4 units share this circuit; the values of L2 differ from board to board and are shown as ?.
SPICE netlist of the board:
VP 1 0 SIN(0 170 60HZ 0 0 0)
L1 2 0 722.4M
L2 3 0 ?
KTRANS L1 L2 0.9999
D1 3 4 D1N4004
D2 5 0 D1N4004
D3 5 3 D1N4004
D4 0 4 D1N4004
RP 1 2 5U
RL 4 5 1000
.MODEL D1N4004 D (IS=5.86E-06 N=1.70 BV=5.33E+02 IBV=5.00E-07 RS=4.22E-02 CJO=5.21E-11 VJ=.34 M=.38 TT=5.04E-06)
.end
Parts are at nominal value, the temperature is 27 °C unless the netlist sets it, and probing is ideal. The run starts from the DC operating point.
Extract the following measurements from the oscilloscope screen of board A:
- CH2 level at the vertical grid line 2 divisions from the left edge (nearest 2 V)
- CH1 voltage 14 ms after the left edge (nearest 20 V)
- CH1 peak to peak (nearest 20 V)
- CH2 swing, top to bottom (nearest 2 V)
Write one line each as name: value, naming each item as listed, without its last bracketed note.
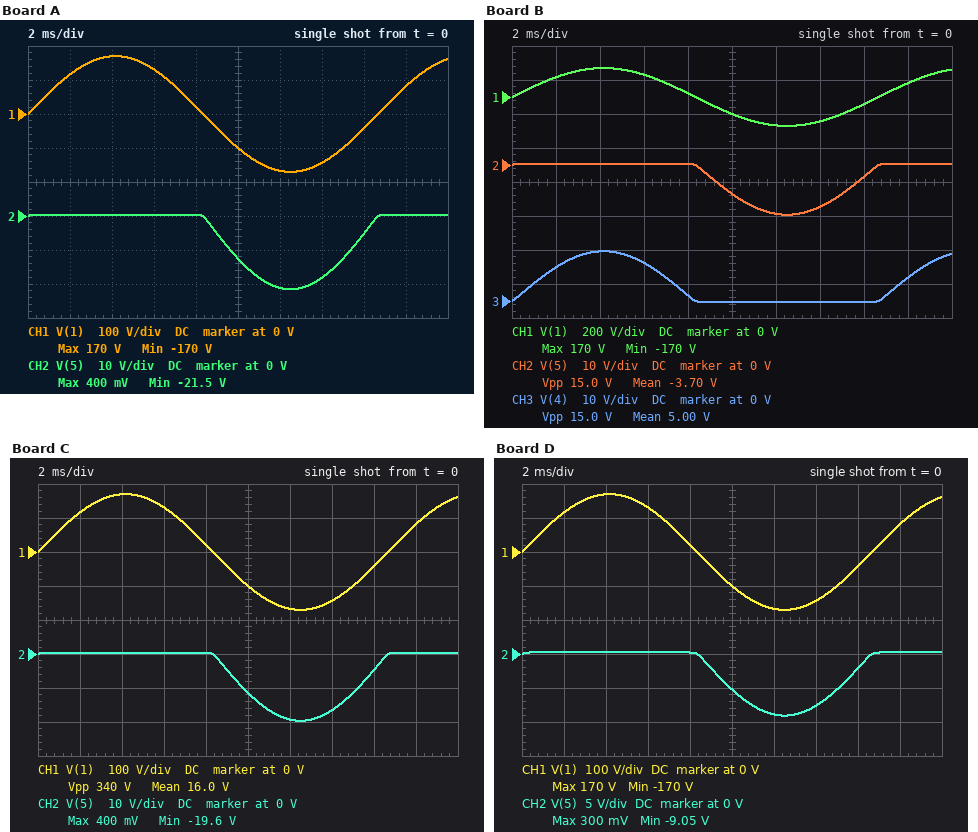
CH2 level at the vertical grid line 2 divisions from the left edge: 0 V
CH1 voltage 14 ms after the left edge: -140 V
CH1 peak to peak: 340 V
CH2 swing, top to bottom: 22 V
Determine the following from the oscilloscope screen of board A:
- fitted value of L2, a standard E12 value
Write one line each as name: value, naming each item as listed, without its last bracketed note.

fitted value of L2, a standard E12 value: 12 mH
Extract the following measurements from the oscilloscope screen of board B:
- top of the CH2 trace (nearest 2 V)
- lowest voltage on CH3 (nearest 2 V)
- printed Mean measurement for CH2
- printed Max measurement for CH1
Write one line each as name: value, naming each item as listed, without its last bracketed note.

top of the CH2 trace: 0 V
lowest voltage on CH3: 0 V
printed Mean measurement for CH2: -3.70 V
printed Max measurement for CH1: 170 V
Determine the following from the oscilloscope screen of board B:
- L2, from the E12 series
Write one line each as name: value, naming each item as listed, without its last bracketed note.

L2, from the E12 series: 5.6 mH
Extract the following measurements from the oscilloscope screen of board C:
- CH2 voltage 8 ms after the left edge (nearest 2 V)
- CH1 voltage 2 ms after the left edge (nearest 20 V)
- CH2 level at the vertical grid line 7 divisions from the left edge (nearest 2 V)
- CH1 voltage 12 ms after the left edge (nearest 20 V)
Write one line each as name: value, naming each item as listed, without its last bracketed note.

CH2 voltage 8 ms after the left edge: 0 V
CH1 voltage 2 ms after the left edge: 120 V
CH2 level at the vertical grid line 7 divisions from the left edge: -16 V
CH1 voltage 12 ms after the left edge: -160 V
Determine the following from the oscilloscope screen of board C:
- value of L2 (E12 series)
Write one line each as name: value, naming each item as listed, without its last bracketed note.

value of L2: 10 mH
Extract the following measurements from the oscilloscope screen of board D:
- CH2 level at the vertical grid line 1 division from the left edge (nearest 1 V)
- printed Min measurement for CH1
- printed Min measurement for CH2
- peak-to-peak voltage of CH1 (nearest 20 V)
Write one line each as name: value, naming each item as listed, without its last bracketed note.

CH2 level at the vertical grid line 1 division from the left edge: 0 V
printed Min measurement for CH1: -170 V
printed Min measurement for CH2: -9.05 V
peak-to-peak voltage of CH1: 340 V
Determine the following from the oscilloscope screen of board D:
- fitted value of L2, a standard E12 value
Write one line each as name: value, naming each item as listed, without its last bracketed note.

fitted value of L2, a standard E12 value: 2.2 mH
